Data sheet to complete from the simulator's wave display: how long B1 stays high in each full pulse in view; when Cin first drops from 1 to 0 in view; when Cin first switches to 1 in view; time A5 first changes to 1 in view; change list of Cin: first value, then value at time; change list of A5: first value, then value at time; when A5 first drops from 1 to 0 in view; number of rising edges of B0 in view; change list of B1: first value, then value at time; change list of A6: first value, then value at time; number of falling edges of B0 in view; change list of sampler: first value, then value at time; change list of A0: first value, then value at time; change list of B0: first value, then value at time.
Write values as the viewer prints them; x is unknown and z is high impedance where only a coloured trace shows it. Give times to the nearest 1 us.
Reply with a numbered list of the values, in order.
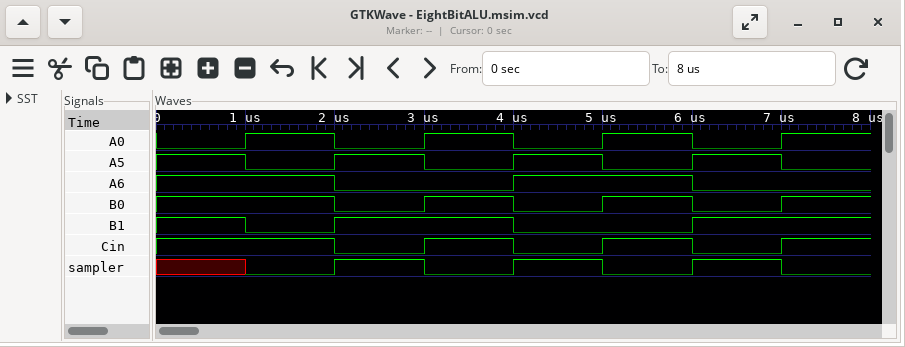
1. 2 us
2. 2 us
3. 3 us
4. 2 us
5. 1, 0 at 2 us, 1 at 3 us, 0 at 4 us, 1 at 5 us, 0 at 6 us, 1 at 7 us
6. 1, 0 at 1 us, 1 at 2 us, 0 at 3 us, 1 at 4 us, 0 at 5 us, 1 at 6 us, 0 at 7 us
7. 1 us
8. 3
9. 1, 0 at 1 us, 1 at 2 us, 0 at 4 us, 1 at 6 us
10. 1, 0 at 2 us, 1 at 4 us, 0 at 6 us
11. 3
12. x, 0 at 1 us, 1 at 2 us, 0 at 3 us, 1 at 4 us, 0 at 5 us, 1 at 6 us, 0 at 7 us
13. 0, 1 at 1 us, 0 at 2 us, 1 at 3 us, 0 at 4 us, 1 at 5 us, 0 at 6 us, 1 at 7 us
14. 1, 0 at 2 us, 1 at 3 us, 0 at 4 us, 1 at 5 us, 0 at 6 us, 1 at 7 us
